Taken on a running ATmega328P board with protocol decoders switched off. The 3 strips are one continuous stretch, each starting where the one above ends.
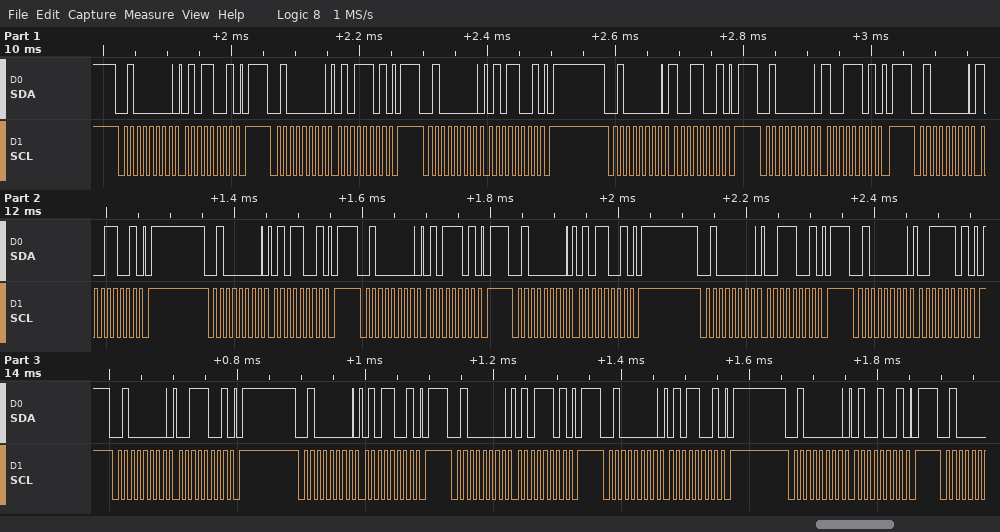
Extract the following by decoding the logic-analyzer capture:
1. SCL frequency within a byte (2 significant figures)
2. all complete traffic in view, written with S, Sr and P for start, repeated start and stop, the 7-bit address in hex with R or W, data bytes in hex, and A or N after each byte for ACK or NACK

100 kHz
S 20W A 59 A P S 20W A 5D A P S 20W A 59 A P S 20W A 99 A P S 20W A 9D A P S 20W A 99 A P S 20W A 59 A P S 20W A 5D A P S 20W A 59 A P S 20W A 39 A P S 20W A 3D A P S 20W A 39 A P S 20W A 59 A P S 20W A 5D A P S 20W A 59 A P S 20W A 49 A P
